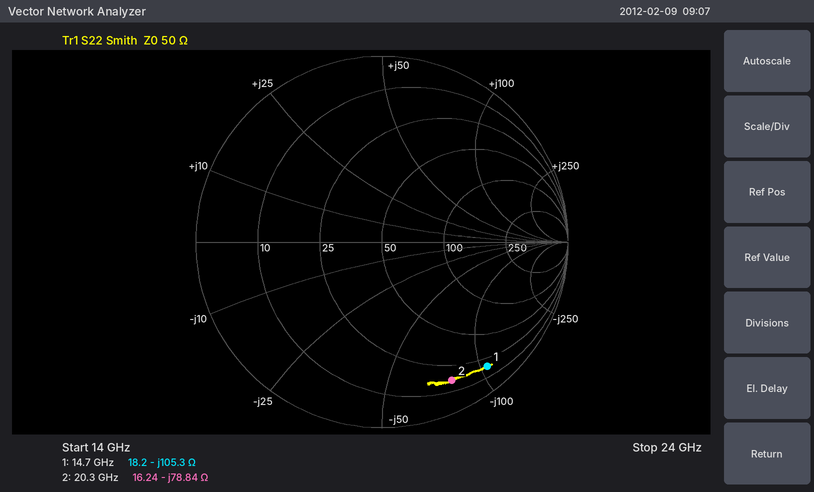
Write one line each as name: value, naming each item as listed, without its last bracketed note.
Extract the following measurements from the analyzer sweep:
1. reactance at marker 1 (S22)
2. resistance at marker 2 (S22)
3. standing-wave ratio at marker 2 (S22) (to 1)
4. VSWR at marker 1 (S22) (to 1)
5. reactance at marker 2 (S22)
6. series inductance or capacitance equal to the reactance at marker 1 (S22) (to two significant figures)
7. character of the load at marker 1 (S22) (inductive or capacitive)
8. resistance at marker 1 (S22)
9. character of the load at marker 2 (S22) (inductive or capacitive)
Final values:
reactance at marker 1: -105.3 Ω
resistance at marker 2: 16.24 Ω
standing-wave ratio at marker 2 (S22): 11
VSWR at marker 1 (S22): 15
reactance at marker 2: -78.84 Ω
series inductance or capacitance equal to the reactance at marker 1 (S22): 100 fF
character of the load at marker 1 (S22): capacitive
resistance at marker 1: 18.2 Ω
character of the load at marker 2 (S22): capacitive
